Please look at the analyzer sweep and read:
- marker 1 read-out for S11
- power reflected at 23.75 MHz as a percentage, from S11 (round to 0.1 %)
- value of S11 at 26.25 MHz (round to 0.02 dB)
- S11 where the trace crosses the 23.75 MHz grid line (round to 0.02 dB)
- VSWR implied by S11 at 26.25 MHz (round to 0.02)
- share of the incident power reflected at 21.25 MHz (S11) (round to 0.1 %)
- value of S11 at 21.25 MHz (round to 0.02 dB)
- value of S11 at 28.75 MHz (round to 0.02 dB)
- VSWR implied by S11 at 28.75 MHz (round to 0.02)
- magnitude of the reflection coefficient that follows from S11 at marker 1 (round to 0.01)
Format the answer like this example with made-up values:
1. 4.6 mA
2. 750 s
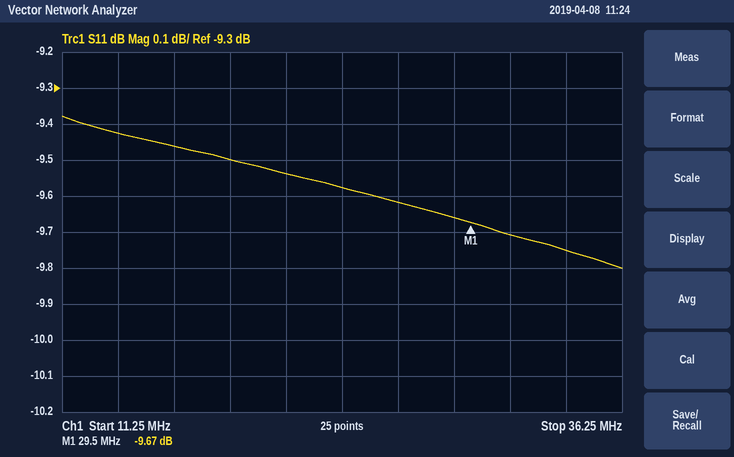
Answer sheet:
1. -9.67 dB
2. 11.0 %
3. -9.62 dB
4. -9.58 dB
5. 1.98
6. 11.1 %
7. -9.54 dB
8. -9.66 dB
9. 1.98
10. 0.33
